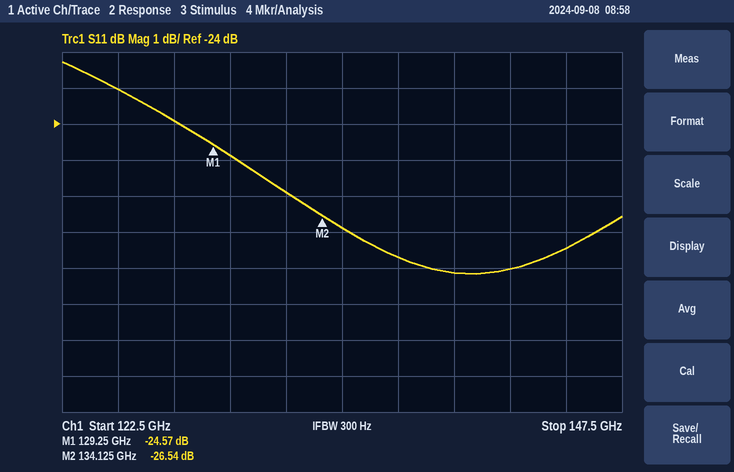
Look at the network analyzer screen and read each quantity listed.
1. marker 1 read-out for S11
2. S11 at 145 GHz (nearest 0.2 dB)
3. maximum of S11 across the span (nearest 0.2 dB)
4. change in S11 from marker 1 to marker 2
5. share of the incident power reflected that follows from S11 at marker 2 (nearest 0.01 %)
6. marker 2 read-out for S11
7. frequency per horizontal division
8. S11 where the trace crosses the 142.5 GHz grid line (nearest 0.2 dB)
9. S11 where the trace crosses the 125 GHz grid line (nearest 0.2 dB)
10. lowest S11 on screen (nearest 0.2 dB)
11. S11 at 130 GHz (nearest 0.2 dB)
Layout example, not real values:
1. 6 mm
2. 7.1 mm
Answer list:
1. -24.57 dB
2. -27.4 dB
3. -22.2 dB
4. -1.97 dB
5. 0.22 %
6. -26.54 dB
7. 2.5 GHz
8. -28.0 dB
9. -23.0 dB
10. -28.2 dB
11. -24.8 dB
